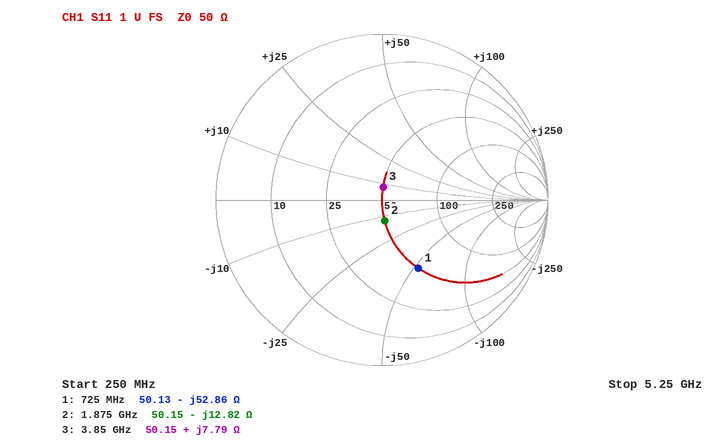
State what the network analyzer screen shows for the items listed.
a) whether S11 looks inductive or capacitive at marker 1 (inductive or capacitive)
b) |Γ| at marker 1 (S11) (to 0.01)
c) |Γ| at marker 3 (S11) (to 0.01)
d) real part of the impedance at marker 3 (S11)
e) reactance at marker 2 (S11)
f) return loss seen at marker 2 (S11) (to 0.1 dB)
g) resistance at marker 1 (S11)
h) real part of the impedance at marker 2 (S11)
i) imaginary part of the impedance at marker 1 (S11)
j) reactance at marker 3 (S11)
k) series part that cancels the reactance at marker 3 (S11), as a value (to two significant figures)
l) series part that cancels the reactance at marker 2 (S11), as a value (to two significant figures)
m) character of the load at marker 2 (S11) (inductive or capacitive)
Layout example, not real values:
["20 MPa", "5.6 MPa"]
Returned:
["capacitive", "0.47", "0.08", "50.15 Ω", "-12.82 Ω", "17.9 dB", "50.13 Ω", "50.15 Ω", "-52.86 Ω", "+7.79 Ω", "5.3 pF", "1.1 nH", "capacitive"]
